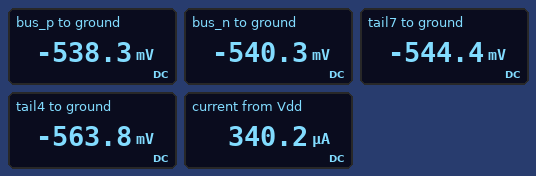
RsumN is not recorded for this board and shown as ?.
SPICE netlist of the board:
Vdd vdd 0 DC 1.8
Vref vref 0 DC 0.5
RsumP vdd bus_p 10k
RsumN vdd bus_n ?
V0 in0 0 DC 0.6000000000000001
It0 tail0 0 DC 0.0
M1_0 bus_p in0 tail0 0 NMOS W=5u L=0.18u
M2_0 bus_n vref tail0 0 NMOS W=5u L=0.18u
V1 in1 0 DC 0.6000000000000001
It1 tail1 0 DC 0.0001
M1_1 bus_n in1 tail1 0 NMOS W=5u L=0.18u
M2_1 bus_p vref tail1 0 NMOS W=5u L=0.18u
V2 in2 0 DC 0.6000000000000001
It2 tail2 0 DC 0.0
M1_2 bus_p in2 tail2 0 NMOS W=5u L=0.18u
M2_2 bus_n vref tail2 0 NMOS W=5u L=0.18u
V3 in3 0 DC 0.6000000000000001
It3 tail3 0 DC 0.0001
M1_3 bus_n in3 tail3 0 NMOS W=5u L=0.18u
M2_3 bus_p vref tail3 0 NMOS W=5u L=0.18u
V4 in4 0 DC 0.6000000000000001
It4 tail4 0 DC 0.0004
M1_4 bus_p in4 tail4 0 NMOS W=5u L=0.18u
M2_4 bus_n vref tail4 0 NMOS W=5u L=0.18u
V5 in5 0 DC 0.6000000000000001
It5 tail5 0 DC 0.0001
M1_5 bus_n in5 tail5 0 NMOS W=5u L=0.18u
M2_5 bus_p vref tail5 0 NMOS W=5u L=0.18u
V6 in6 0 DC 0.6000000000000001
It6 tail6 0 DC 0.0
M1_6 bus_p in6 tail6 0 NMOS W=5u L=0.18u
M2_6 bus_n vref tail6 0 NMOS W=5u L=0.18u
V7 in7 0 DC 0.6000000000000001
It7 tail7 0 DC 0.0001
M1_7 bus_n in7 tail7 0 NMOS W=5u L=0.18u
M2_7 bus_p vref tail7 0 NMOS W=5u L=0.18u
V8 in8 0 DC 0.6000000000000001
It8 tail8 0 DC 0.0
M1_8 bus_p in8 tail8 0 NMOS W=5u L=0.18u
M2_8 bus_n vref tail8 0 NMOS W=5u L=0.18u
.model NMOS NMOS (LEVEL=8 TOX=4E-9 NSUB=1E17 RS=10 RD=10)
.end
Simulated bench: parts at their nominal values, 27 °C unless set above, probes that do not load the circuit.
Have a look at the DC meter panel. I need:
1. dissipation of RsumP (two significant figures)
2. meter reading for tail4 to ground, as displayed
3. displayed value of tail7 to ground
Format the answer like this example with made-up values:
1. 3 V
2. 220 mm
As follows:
1. 550 µW
2. -563.8 mV
3. -544.4 mV
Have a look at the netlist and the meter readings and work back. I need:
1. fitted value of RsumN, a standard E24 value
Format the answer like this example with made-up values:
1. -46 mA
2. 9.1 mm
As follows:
1. 22 kΩ
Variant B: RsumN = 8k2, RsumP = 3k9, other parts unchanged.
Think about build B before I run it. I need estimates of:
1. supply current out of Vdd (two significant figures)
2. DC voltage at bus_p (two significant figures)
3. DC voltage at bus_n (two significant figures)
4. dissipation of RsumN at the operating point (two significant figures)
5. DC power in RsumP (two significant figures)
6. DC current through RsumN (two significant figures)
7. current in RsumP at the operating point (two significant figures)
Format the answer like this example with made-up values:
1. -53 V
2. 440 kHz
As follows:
1. 800 µA
2. -310 mV
3. -320 mV
4. 550 µW
5. 1.1 mW
6. 260 µA
7. 540 µA
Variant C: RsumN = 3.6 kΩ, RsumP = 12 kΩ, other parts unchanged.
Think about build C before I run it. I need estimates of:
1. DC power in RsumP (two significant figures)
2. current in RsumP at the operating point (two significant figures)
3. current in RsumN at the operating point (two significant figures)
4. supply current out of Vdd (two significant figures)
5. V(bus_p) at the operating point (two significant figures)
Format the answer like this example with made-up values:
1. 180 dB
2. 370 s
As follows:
1. 410 µW
2. 180 µA
3. 610 µA
4. 800 µA
5. -410 mV
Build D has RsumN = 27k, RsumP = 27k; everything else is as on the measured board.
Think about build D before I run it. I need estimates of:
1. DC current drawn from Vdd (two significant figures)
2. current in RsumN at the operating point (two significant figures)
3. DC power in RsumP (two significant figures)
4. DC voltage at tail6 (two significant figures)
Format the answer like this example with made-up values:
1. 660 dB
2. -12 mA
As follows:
1. 170 µA
2. 87 µA
3. 200 µW
4. -550 mV
